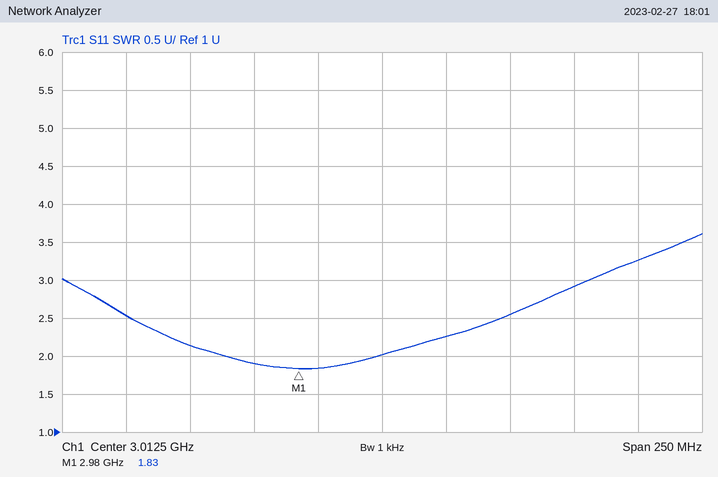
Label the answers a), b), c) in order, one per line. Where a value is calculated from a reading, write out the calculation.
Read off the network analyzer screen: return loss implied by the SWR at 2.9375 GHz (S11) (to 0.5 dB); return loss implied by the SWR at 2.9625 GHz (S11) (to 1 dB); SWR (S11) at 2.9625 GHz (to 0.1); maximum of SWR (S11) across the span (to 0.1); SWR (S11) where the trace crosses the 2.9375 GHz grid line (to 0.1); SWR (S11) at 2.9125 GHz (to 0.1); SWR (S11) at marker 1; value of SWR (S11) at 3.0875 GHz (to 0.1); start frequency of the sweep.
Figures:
a) −20 log10((2.1 − 1)/(2.1 + 1)) ≈ 9.0 dB
b) −20 log10((1.9 − 1)/(1.9 + 1)) ≈ 10 dB
c) 1.9
d) 3.6
e) 2.1
f) 2.5
g) 1.83
h) 2.9
i) 2.8875 GHz
